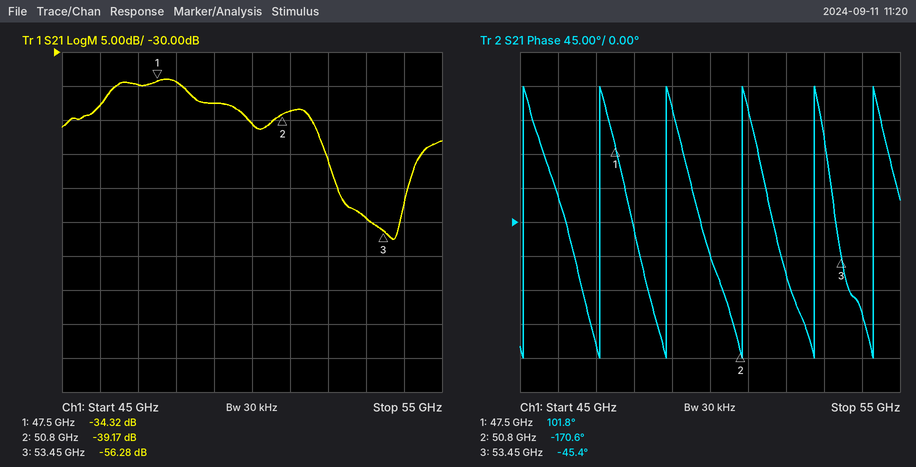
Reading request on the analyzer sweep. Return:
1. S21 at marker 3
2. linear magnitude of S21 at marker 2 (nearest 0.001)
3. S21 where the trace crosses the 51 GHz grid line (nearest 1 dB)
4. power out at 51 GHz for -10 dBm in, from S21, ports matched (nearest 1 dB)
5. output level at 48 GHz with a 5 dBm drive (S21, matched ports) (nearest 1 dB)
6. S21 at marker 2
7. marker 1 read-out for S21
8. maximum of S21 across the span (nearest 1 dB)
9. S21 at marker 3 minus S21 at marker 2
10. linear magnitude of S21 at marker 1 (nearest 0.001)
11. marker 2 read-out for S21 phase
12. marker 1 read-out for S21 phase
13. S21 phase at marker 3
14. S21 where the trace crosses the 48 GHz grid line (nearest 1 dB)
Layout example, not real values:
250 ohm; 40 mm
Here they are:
-56.28 dB; 0.011; -39 dB; -49 dBm; -29 dBm; -39.17 dB; -34.32 dB; -34 dB; -17.11 dB; 0.019; -170.6°; 101.8°; -45.4°; -34 dB
